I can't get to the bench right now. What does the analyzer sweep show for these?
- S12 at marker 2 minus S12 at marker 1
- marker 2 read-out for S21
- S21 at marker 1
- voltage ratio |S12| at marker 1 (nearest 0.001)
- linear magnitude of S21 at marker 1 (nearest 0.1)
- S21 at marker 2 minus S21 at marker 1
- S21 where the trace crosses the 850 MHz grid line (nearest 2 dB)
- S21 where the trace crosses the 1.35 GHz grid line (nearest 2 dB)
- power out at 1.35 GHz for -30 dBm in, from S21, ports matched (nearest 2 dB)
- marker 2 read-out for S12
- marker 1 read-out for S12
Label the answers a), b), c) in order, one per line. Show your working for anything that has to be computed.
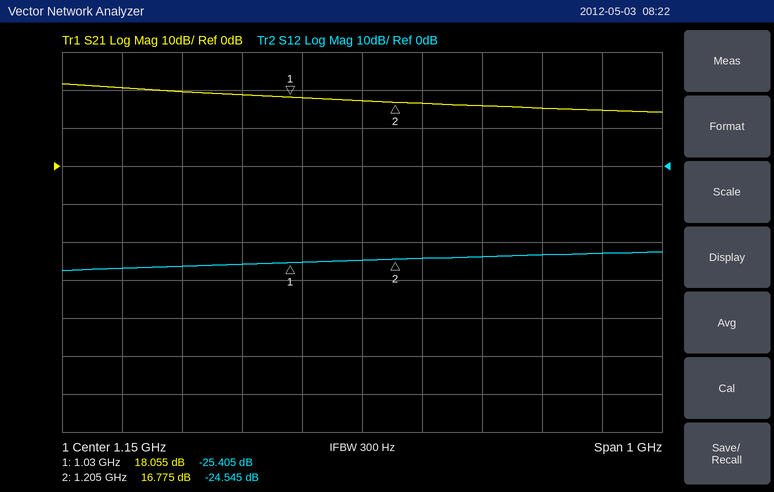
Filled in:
a) -24.545 − (-25.405) = 0.860 dB
b) 16.775 dB
c) 18.055 dB
d) 10^(-25.405/20) ≈ 0.054
e) 10^(18.055/20) ≈ 8.0
f) 16.775 − (18.055) = -1.280 dB
g) 20 dB
h) 16 dB
i) -30 dBm + (16 dB) = -14 dBm
j) -24.545 dB
k) -25.405 dB
